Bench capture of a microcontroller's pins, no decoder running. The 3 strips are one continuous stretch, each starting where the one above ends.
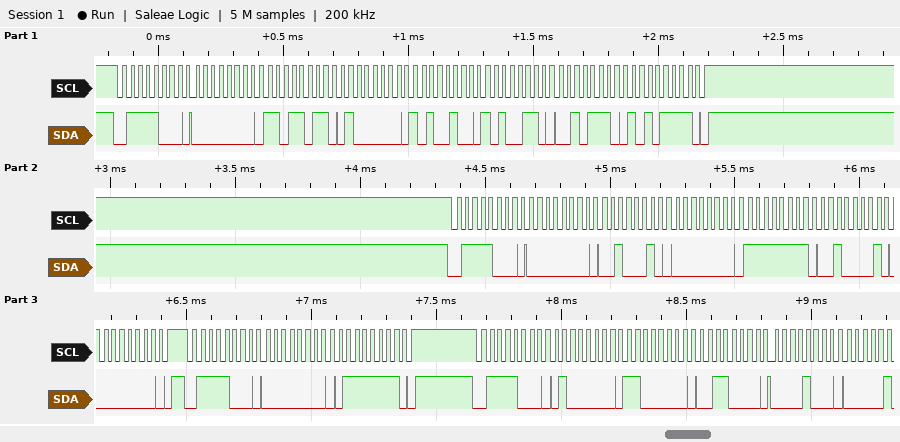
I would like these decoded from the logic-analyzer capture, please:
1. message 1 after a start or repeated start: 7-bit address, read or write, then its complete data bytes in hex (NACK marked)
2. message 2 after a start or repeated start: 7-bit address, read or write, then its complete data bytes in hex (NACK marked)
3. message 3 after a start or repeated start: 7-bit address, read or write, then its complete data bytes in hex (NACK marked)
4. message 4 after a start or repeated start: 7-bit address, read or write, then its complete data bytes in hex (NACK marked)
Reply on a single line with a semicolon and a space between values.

0x3C write: 00 DB 40 A4 A6 2E AF; 0x3C write: 00 22 00 FF 21 00; 0x3C write: 00 7F; 0x3C write: 40 C0 30 08
